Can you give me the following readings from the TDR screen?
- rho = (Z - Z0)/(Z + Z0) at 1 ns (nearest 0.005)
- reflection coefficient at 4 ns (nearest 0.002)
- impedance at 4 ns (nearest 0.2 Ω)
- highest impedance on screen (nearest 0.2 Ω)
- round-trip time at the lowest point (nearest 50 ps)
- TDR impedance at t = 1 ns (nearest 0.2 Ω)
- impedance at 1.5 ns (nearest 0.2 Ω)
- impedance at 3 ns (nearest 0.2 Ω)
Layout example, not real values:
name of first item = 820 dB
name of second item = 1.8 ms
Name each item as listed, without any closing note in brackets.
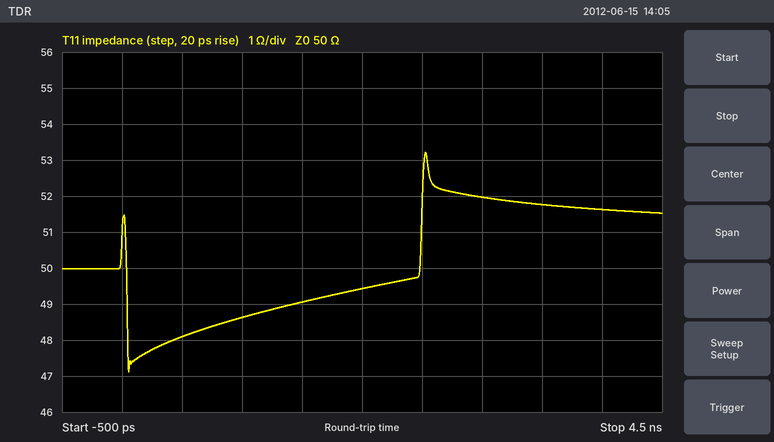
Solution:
rho = (Z - Z0)/(Z + Z0) at 1 ns = -0.015
reflection coefficient at 4 ns = +0.016
impedance at 4 ns = 51.6 Ω
highest impedance on screen = 53.2 Ω
round-trip time at the lowest point = 50 ps
TDR impedance at t = 1 ns = 48.6 Ω
impedance at 1.5 ns = 49.0 Ω
impedance at 3 ns = 52.0 Ω
